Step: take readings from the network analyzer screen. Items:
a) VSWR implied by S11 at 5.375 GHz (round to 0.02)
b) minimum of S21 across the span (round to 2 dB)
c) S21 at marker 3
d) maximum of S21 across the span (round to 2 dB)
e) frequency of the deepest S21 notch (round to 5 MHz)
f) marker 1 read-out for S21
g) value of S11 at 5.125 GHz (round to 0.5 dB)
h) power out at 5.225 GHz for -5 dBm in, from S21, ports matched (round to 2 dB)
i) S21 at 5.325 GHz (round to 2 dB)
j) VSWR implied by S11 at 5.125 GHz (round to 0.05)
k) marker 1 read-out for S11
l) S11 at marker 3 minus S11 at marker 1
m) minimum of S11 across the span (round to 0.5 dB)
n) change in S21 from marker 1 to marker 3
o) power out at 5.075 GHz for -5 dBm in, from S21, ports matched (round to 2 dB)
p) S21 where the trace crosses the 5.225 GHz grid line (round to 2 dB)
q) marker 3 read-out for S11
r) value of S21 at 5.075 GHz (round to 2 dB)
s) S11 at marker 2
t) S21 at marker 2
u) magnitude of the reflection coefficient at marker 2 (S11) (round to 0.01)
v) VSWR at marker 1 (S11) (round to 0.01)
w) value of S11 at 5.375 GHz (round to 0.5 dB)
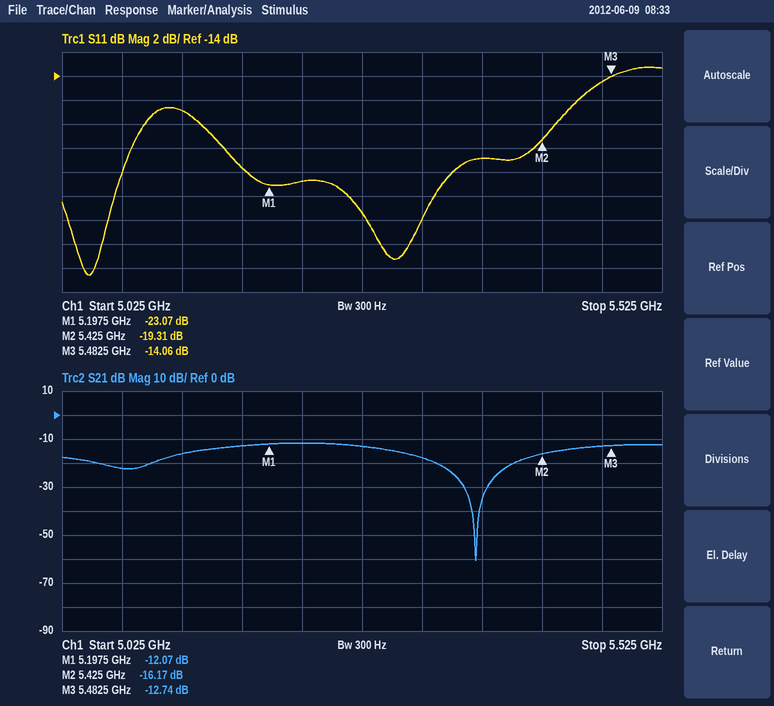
1.20
-60 dB
-12.74 dB
-12 dB
5.370 GHz
-12.07 dB
-17.0 dB
-16 dBm
-18 dB
1.35
-23.07 dB
9.01 dB
-30.5 dB
-0.67 dB
-28 dBm
-12 dB
-14.06 dB
-22 dB
-19.31 dB
-16.17 dB
0.11
1.15
-21.0 dB
